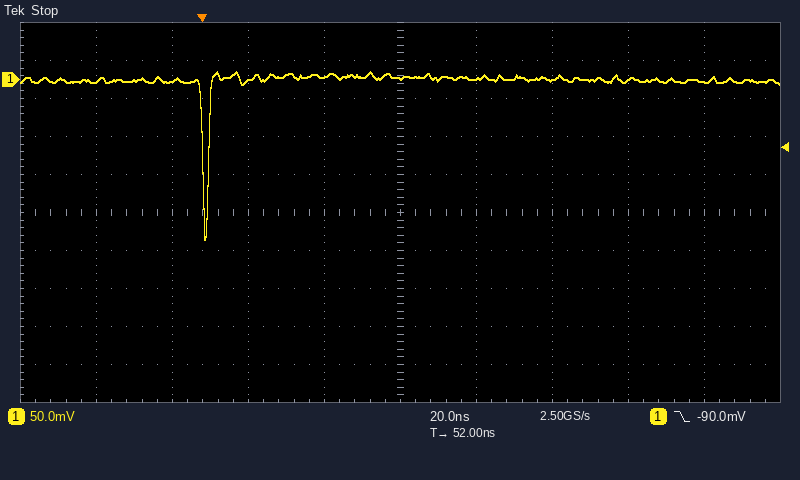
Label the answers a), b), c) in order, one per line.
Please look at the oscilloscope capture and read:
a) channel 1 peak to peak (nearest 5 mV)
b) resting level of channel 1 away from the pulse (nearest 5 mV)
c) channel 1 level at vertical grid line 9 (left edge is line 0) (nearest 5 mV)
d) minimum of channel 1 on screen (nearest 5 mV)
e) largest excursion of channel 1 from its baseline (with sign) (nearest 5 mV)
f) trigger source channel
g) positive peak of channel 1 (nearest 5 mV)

a) 220 mV
b) 0 mV
c) -5 mV
d) -210 mV
e) -210 mV
f) channel 1
g) 10 mV
